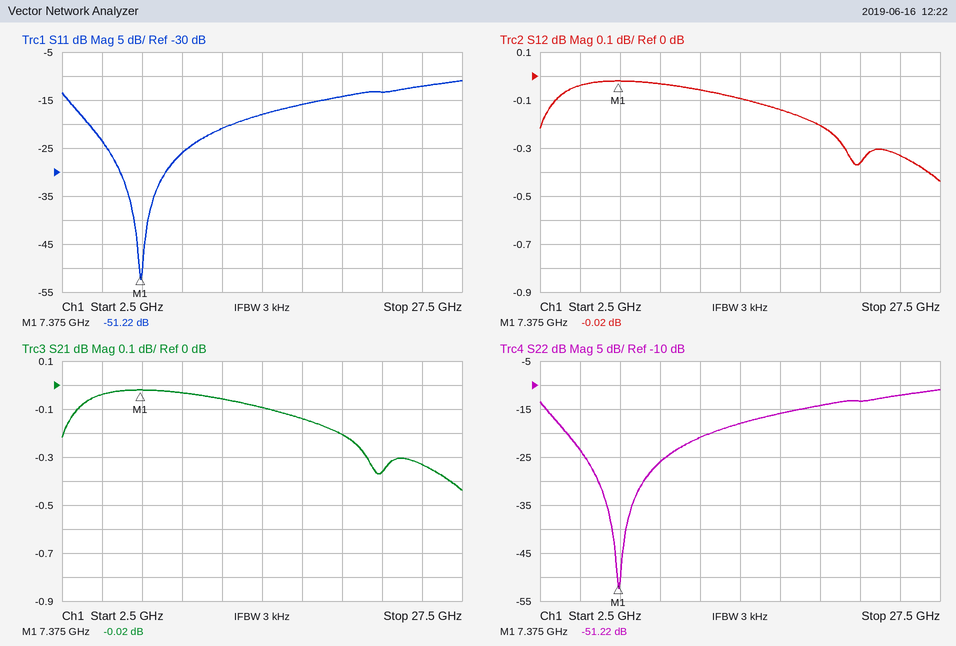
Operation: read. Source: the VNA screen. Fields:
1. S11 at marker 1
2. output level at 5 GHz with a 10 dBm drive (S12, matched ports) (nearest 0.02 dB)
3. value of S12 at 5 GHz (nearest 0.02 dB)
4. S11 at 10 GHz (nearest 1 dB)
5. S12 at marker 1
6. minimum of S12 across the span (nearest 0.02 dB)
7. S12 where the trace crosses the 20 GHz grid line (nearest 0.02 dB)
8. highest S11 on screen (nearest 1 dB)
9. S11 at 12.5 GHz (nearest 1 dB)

-51.22 dB
9.96 dBm
-0.04 dB
-26 dB
-0.02 dB
-0.44 dB
-0.20 dB
-11 dB
-21 dB
